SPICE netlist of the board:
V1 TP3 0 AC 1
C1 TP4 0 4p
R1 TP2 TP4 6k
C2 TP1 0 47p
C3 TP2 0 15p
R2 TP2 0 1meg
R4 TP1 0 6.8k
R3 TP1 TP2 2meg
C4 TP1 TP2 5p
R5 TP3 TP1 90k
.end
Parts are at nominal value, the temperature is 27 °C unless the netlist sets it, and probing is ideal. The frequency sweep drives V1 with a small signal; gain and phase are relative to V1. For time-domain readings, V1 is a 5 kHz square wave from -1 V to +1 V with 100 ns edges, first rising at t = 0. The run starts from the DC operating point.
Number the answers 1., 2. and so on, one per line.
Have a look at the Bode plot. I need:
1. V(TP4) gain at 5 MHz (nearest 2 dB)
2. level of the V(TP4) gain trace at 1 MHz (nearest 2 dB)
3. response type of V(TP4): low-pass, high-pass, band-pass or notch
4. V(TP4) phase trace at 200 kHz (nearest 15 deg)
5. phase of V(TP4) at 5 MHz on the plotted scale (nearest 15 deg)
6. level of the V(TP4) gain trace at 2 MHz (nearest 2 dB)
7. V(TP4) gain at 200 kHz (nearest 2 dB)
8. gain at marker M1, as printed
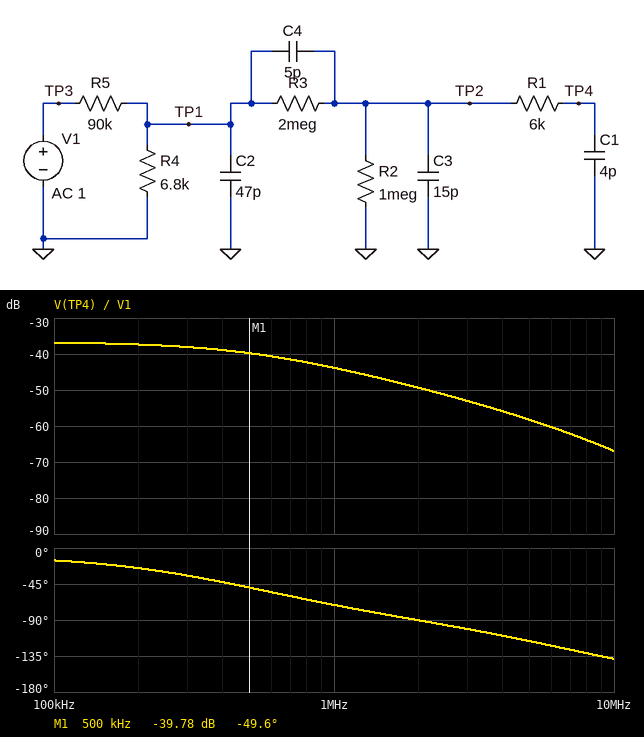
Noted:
1. -58 dB
2. -44 dB
3. low-pass
4. -30 deg
5. -120 deg
6. -50 dB
7. -38 dB
8. -39.78 dB
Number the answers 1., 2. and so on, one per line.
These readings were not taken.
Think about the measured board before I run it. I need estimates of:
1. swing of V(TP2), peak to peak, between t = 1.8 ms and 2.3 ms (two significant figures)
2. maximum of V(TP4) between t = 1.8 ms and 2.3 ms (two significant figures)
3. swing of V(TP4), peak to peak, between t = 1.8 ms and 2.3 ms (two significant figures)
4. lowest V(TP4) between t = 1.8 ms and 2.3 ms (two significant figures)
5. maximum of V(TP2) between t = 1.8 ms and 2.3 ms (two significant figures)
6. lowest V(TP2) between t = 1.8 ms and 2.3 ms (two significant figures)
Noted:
1. 47 mV
2. 23 mV
3. 47 mV
4. -23 mV
5. 23 mV
6. -23 mV
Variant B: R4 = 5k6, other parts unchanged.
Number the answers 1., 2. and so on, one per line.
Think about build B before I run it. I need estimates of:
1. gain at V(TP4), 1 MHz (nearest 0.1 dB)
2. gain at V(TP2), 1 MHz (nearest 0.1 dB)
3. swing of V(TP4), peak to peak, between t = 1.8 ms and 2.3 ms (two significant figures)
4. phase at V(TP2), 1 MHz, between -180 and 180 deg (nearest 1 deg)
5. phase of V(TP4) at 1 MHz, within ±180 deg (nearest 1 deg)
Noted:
1. -44.2 dB
2. -44.1 dB
3. 39 mV
4. -58 deg
5. -67 deg
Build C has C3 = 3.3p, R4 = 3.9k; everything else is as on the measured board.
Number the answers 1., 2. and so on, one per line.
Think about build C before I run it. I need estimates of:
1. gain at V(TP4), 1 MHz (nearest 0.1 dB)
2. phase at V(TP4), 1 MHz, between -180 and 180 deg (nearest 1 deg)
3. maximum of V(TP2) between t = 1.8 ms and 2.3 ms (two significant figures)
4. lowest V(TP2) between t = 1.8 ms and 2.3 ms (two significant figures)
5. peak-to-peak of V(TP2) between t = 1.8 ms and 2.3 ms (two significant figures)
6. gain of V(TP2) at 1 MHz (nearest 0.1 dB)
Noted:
1. -39.3 dB
2. -55 deg
3. 19 mV
4. -19 mV
5. 38 mV
6. -39.2 dB
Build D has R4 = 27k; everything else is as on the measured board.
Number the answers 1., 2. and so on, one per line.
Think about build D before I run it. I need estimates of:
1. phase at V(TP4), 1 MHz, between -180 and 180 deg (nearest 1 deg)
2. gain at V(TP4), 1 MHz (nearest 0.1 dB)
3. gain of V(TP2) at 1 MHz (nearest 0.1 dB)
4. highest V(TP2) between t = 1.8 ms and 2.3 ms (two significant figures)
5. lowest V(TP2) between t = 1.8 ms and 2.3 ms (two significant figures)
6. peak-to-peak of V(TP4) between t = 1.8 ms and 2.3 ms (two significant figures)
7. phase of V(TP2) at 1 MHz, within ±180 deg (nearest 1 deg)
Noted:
1. -89 deg
2. -43.0 dB
3. -42.9 dB
4. 76 mV
5. -76 mV
6. 150 mV
7. -80 deg
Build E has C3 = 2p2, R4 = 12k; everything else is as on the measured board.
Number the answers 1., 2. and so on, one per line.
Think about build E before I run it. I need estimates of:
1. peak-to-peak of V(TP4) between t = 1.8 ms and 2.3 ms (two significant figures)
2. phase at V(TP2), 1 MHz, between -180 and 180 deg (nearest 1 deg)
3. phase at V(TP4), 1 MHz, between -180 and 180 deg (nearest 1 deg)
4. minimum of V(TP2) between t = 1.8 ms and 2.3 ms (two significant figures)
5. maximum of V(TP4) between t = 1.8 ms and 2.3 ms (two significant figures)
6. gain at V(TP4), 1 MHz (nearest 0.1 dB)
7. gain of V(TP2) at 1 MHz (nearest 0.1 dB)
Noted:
1. 120 mV
2. -70 deg
3. -78 deg
4. -59 mV
5. 59 mV
6. -36.4 dB
7. -36.3 dB
